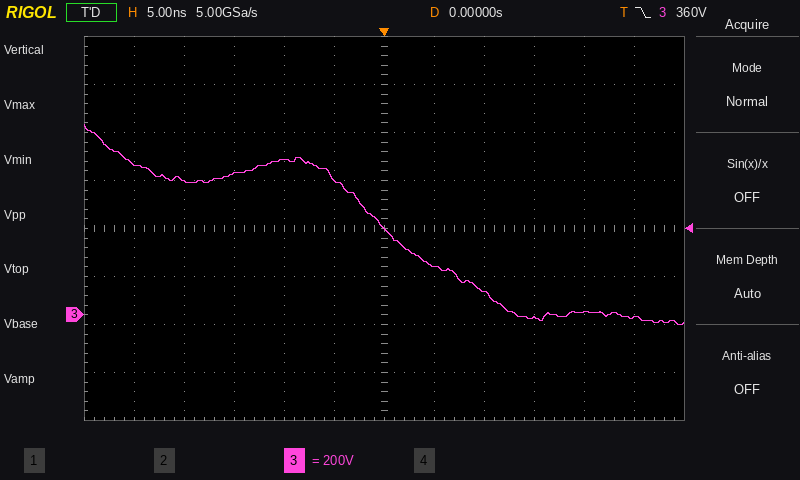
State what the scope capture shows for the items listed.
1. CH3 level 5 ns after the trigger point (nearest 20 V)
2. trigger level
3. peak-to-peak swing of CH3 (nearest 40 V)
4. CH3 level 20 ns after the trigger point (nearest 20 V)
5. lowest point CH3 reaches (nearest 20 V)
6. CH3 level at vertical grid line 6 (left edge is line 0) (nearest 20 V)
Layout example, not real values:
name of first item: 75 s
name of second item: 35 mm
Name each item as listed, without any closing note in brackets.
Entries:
CH3 level 5 ns after the trigger point: 200 V
trigger level: 360 V
peak-to-peak swing of CH3: 840 V
CH3 level 20 ns after the trigger point: 20 V
lowest point CH3 reaches: -40 V
CH3 level at vertical grid line 6 (left edge is line 0): 360 V
